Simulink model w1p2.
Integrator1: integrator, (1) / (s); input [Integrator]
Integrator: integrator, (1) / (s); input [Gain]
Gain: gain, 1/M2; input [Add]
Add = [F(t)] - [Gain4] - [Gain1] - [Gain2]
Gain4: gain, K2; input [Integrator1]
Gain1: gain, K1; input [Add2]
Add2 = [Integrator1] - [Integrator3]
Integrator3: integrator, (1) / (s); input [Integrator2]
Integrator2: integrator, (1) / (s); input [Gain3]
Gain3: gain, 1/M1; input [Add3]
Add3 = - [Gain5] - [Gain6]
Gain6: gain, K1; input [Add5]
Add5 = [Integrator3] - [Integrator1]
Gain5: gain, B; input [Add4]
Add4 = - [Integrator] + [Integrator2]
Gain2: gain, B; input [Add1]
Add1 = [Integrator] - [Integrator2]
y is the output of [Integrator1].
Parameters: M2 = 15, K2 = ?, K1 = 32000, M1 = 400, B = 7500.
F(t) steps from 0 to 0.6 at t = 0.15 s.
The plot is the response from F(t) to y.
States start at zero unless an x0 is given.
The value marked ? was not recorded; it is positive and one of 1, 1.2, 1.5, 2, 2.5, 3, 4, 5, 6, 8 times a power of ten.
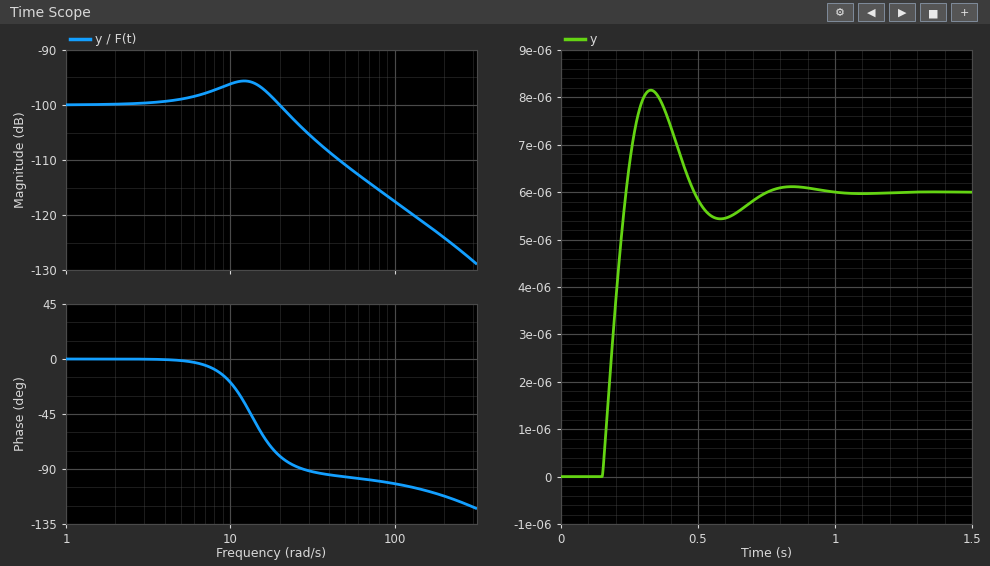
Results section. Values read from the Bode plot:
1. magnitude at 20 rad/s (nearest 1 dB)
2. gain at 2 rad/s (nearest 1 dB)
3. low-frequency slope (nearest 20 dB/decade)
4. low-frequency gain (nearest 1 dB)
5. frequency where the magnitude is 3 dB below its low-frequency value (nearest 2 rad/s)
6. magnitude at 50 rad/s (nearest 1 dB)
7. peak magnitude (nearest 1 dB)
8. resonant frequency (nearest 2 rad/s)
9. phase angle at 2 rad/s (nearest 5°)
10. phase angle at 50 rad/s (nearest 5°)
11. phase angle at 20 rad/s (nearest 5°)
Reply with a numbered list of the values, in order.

1. -100 dB
2. -100 dB
3. 0 dB/decade
4. -100 dB
5. 24 rad/s
6. -111 dB
7. -96 dB
8. 12 rad/s
9. 0°
10. -95°
11. -80°
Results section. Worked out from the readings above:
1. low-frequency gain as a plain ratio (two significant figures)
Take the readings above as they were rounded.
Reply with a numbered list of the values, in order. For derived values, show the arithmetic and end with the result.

1. 10^(-100 / 20) = 0.000010
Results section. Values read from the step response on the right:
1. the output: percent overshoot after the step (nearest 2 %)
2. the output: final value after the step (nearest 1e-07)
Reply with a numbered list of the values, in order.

1. 36 %
2. 0.0000060
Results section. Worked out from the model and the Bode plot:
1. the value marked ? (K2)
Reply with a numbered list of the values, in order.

1. 100000
